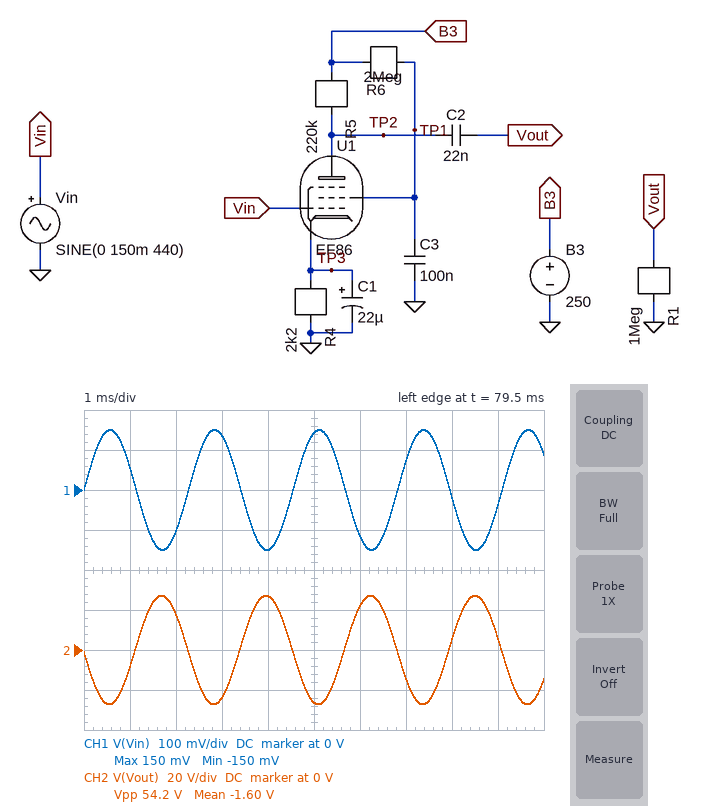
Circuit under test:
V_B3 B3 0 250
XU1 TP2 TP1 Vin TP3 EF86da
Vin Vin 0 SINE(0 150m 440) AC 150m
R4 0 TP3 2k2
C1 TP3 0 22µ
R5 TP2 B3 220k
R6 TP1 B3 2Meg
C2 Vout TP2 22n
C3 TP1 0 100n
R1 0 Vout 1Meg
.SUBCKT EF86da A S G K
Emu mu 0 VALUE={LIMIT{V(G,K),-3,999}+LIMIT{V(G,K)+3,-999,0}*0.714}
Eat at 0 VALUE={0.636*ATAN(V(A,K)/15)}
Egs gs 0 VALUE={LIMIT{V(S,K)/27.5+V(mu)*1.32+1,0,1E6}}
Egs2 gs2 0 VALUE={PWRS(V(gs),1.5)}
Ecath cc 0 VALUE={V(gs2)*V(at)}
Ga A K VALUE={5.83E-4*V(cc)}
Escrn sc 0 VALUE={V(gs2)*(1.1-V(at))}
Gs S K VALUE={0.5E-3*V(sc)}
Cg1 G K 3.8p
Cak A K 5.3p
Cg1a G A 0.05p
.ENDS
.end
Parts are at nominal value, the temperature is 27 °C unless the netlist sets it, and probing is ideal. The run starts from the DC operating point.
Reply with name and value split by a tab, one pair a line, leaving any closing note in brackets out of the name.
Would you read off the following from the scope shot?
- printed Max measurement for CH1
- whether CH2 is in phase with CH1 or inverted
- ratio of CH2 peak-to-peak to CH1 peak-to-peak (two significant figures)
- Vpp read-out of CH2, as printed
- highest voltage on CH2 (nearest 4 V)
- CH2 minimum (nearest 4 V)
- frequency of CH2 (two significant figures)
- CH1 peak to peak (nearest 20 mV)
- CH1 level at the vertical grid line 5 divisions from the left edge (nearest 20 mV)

printed Max measurement for CH1	150 mV
whether CH2 is in phase with CH1 or inverted	inverted
ratio of CH2 peak-to-peak to CH1 peak-to-peak	180
Vpp read-out of CH2, as printed	54.2 V
highest voltage on CH2	28 V
CH2 minimum	-28 V
frequency of CH2	440 Hz
CH1 peak to peak	300 mV
CH1 level at the vertical grid line 5 divisions from the left edge	140 mV
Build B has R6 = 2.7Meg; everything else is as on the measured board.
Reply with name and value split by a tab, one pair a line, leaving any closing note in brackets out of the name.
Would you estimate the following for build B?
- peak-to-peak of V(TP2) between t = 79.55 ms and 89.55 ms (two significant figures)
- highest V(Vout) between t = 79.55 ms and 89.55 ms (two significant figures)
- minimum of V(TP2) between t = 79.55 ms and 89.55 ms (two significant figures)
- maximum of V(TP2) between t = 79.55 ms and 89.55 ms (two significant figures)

peak-to-peak of V(TP2) between t = 79.55 ms and 89.55 ms	53 V
highest V(Vout) between t = 79.55 ms and 89.55 ms	26 V
minimum of V(TP2) between t = 79.55 ms and 89.55 ms	120 V
maximum of V(TP2) between t = 79.55 ms and 89.55 ms	170 V
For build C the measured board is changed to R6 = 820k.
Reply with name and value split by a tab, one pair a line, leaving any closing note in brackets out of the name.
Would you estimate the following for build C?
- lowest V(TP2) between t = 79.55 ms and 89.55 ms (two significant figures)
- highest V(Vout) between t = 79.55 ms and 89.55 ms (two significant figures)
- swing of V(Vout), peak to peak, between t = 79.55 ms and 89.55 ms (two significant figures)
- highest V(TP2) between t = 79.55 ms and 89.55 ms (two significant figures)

lowest V(TP2) between t = 79.55 ms and 89.55 ms	52 V
highest V(Vout) between t = 79.55 ms and 89.55 ms	25 V
swing of V(Vout), peak to peak, between t = 79.55 ms and 89.55 ms	47 V
highest V(TP2) between t = 79.55 ms and 89.55 ms	99 V
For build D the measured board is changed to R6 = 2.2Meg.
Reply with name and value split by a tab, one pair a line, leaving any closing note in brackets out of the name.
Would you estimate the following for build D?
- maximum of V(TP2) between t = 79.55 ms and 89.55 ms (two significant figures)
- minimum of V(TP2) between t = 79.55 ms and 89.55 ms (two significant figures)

maximum of V(TP2) between t = 79.55 ms and 89.55 ms	160 V
minimum of V(TP2) between t = 79.55 ms and 89.55 ms	100 V
